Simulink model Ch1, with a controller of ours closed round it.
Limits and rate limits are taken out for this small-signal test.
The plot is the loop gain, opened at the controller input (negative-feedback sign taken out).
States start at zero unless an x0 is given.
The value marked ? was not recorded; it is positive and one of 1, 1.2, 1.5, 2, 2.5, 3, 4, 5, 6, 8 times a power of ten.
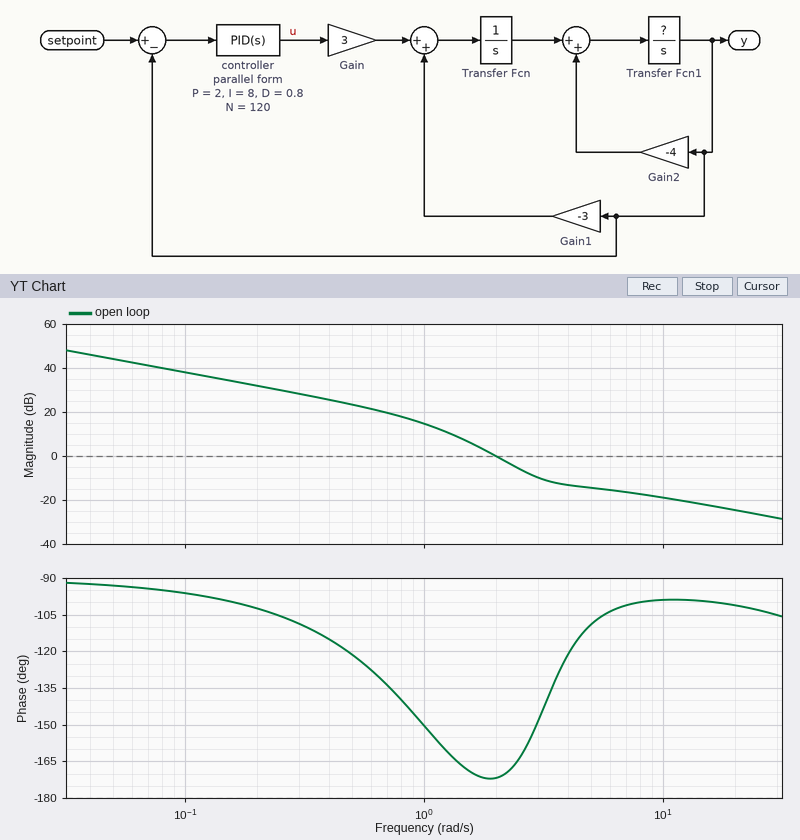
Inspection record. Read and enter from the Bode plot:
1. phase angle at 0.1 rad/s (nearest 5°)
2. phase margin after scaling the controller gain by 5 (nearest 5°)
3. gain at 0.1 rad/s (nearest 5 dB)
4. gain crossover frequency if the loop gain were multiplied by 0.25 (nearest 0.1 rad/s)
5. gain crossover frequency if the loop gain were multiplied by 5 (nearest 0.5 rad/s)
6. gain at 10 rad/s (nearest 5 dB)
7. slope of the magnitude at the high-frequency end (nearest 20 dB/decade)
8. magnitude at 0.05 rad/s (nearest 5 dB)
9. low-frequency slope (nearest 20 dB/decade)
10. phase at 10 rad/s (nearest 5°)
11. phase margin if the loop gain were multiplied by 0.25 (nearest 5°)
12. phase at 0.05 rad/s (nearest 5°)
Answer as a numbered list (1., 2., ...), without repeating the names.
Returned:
1. -95°
2. 65°
3. 40 dB
4. 1.2 rad/s
5. 4.5 rad/s
6. -20 dB
7. -20 dB/decade
8. 45 dB
9. -20 dB/decade
10. -100°
11. 20°
12. -95°
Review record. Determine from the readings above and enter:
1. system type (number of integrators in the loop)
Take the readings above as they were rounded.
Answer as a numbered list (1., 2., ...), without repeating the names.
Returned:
1. 1
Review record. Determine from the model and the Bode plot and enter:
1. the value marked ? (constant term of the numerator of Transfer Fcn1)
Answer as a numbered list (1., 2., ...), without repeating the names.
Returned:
1. 0.5
